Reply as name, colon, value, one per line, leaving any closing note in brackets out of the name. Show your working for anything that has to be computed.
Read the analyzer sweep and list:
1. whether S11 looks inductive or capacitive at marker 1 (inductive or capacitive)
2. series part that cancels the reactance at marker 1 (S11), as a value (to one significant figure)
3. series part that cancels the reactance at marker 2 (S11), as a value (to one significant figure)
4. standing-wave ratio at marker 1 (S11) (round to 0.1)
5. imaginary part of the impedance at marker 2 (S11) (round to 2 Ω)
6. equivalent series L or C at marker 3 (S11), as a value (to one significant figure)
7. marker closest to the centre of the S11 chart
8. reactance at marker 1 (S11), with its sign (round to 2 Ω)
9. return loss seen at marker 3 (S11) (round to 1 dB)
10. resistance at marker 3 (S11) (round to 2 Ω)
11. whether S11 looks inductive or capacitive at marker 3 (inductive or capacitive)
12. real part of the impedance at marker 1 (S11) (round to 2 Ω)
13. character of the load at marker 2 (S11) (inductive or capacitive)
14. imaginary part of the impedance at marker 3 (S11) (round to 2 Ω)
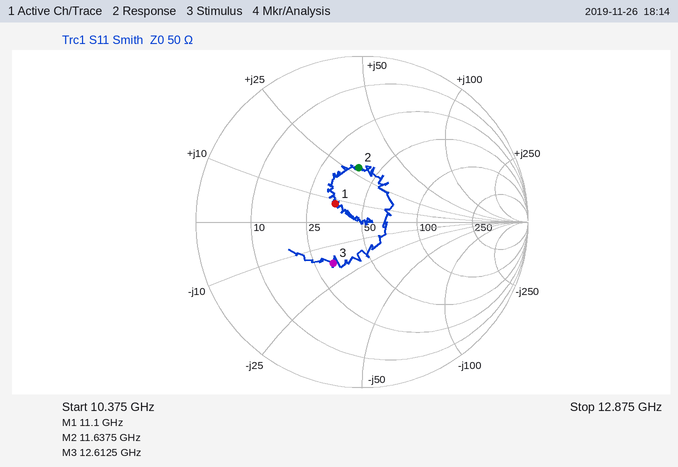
whether S11 looks inductive or capacitive at marker 1: inductive
series part that cancels the reactance at marker 1 (S11), as a value: C = 1/(2π × 11.1 GHz × 8 Ω) ≈ 2 pF
series part that cancels the reactance at marker 2 (S11), as a value: C = 1/(2π × 11.6375 GHz × 28 Ω) ≈ 488 fF, so 500 fF to one significant figure
standing-wave ratio at marker 1 (S11): 1.5
imaginary part of the impedance at marker 2 (S11): +28 Ω
equivalent series L or C at marker 3 (S11), as a value: C = 1/(2π × 12.6125 GHz × 18 Ω) ≈ 701 fF, so 700 fF to one significant figure
marker closest to the centre of the S11 chart: marker 1
reactance at marker 1 (S11), with its sign: +8 Ω
return loss seen at marker 3 (S11): 10 dB
resistance at marker 3 (S11): 32 Ω
whether S11 looks inductive or capacitive at marker 3: capacitive
real part of the impedance at marker 1 (S11): 36 Ω
character of the load at marker 2 (S11): inductive
imaginary part of the impedance at marker 3 (S11): -18 Ω
